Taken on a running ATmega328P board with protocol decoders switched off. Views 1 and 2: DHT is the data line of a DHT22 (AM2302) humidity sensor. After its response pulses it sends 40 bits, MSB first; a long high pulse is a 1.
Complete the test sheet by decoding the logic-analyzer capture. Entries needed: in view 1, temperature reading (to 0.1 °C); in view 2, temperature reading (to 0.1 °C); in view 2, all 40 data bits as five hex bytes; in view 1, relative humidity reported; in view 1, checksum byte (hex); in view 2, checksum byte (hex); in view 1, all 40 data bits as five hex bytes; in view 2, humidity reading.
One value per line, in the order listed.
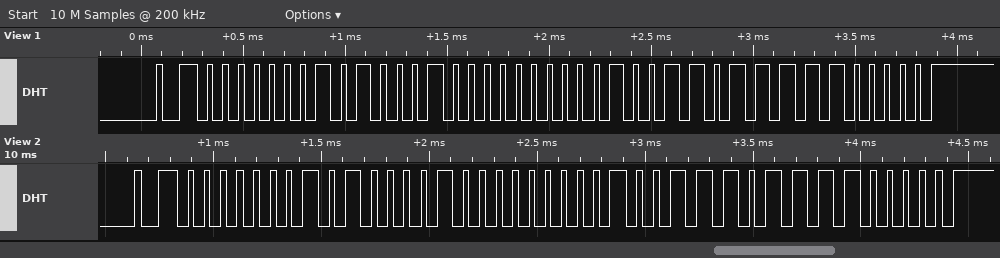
15.5 °C
15.7 °C
01 42 00 9D E0
32.4 %
0xE0
0xE0
01 44 00 9B E0
32.2 %
